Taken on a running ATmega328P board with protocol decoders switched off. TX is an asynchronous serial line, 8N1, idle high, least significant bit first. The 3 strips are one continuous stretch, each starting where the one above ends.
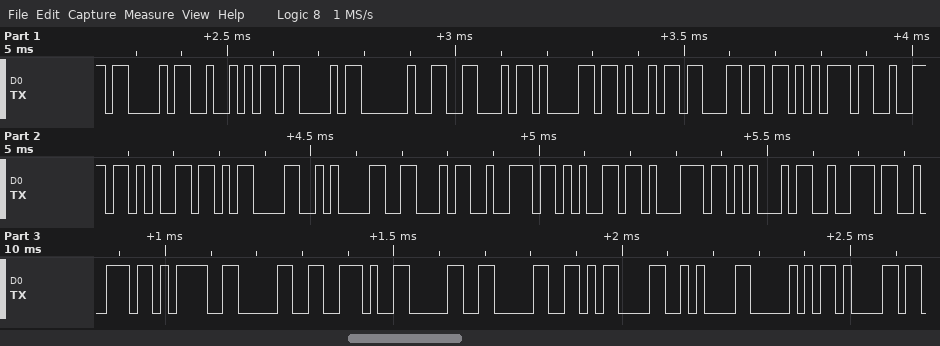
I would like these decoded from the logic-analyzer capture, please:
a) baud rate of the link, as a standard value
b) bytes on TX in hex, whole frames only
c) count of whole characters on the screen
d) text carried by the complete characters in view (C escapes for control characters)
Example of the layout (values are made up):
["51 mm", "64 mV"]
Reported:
["57600 baud", "0x43 0x52 0x43 0x20 0x46 0x61 0x69 0x6C 0x75 0x72 0x65 0x0D 0x0A 0x46 0x72 0x65 0x71 0x45 0x72 0x72 0x3D 0x30 0x2E 0x30 0x30 0x0D 0x0A 0x50 0x61", "29", "\"CRC Failure\\r\\nFreqErr=0.00\\r\\nPa\""]
